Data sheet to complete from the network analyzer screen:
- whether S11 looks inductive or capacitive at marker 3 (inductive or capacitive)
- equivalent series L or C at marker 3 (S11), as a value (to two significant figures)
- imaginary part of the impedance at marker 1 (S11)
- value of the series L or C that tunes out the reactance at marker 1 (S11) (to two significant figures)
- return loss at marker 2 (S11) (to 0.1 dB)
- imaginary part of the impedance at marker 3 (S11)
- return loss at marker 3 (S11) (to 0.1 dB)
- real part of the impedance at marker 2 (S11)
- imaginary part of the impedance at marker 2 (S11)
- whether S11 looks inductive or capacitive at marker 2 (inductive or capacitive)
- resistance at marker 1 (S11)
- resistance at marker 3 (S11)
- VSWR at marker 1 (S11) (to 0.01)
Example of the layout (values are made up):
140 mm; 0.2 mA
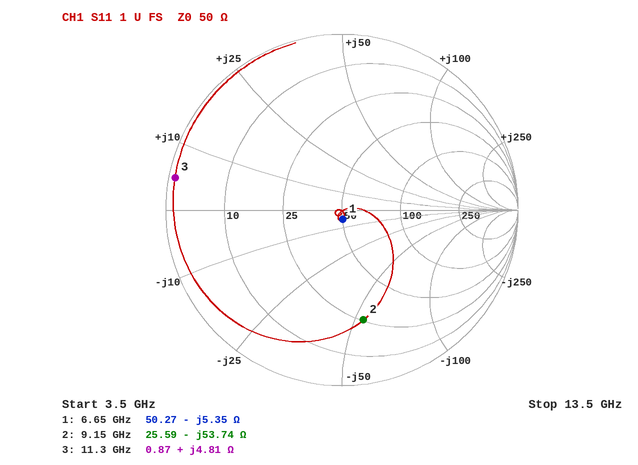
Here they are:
inductive; 68 pH; -5.35 Ω; 130 pH; 3.9 dB; +4.81 Ω; 0.3 dB; 25.59 Ω; -53.74 Ω; capacitive; 50.27 Ω; 0.87 Ω; 1.11
